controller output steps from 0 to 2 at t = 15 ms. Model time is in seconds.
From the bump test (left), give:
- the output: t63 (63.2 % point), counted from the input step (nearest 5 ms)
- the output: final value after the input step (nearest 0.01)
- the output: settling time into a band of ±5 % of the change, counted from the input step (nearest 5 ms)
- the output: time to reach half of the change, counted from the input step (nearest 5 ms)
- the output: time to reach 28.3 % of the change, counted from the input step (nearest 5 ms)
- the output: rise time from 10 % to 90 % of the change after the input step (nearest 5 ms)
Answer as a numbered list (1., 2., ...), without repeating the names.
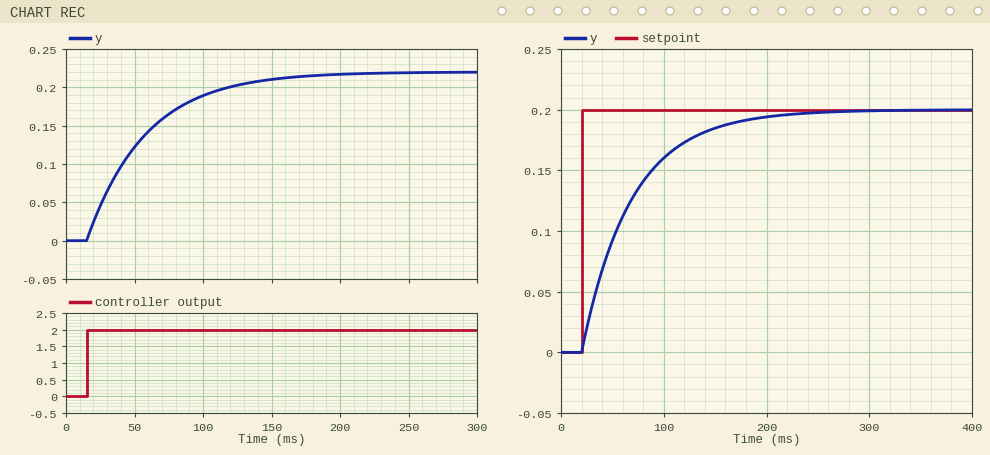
1. 45 ms
2. 0.22
3. 130 ms
4. 30 ms
5. 15 ms
6. 95 ms
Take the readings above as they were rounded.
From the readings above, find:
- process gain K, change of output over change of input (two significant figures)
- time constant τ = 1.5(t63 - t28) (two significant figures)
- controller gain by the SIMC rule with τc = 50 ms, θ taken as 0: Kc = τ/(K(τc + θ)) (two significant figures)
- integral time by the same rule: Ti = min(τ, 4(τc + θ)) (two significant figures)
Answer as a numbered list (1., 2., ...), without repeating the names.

1. 0.11
2. 45 ms
3. 8.2
4. 45 ms
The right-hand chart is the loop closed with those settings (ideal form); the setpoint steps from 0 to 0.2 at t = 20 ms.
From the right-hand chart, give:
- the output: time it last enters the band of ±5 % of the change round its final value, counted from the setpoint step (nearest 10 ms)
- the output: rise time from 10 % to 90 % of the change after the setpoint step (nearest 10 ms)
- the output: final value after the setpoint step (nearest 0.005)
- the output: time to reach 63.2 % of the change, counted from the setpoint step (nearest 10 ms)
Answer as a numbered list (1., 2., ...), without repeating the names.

1. 150 ms
2. 110 ms
3. 0.200
4. 50 ms
